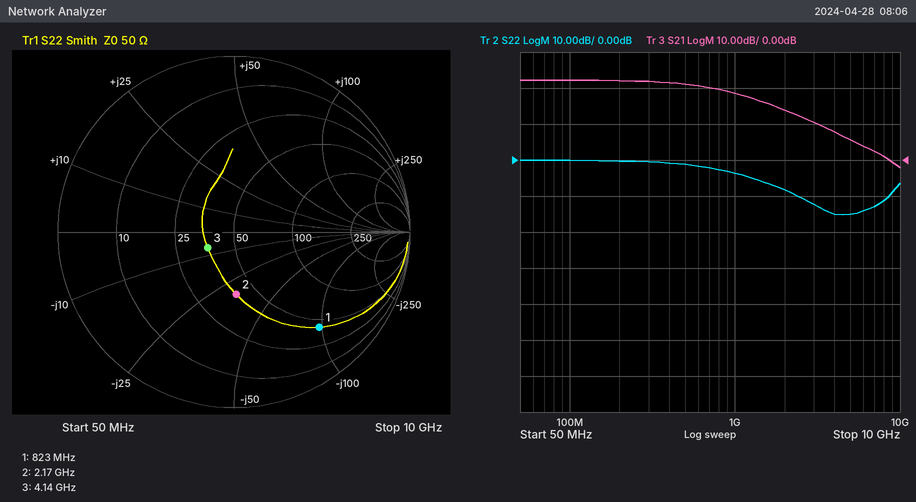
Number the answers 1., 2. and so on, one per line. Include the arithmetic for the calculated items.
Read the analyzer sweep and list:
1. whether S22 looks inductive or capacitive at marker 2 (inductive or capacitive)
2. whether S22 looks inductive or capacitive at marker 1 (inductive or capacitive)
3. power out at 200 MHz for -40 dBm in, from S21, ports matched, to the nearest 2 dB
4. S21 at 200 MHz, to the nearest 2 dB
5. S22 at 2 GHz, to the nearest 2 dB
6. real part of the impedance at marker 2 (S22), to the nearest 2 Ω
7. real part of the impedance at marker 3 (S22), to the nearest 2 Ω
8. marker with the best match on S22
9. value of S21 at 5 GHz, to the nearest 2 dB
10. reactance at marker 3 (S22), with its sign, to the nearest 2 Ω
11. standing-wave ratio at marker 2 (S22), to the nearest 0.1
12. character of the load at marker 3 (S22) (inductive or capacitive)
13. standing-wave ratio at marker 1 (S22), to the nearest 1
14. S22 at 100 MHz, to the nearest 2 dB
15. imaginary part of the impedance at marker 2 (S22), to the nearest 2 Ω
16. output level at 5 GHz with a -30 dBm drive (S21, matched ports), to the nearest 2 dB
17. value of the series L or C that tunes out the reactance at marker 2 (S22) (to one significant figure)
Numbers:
1. capacitive
2. capacitive
3. -40 dBm + (22 dB) = -18 dBm
4. 22 dB
5. -8 dB
6. 40 Ω
7. 36 Ω
8. marker 3
9. 6 dB
10. -6 Ω
11. 2.1
12. capacitive
13. 6
14. 0 dB
15. -32 Ω
16. -30 dBm + (6 dB) = -24 dBm
17. L = 32 Ω/(2π × 2.17 GHz) ≈ 2 nH
